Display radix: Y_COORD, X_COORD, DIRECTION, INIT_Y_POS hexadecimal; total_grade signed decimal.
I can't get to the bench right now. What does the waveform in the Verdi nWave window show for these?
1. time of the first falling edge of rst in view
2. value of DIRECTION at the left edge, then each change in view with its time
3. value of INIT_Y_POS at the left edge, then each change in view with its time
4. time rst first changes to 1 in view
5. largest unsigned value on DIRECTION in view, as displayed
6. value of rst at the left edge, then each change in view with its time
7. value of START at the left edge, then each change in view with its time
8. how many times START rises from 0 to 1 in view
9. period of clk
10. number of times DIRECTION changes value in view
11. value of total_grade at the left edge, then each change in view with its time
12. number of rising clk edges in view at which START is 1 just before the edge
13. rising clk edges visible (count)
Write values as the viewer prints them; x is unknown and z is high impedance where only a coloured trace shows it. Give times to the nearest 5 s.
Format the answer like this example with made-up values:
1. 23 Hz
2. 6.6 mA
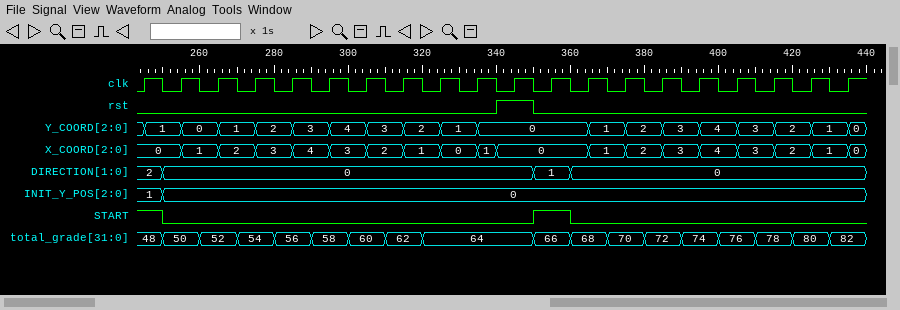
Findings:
1. 350 s
2. 2, 0 at 250 s, 1 at 350 s, 0 at 360 s
3. 1, 0 at 250 s
4. 340 s
5. 2
6. 0, 1 at 340 s, 0 at 350 s
7. 1, 0 at 250 s, 1 at 350 s, 0 at 360 s
8. 1
9. 10 s
10. 3
11. 48, 50 at 250 s, 52 at 260 s, 54 at 270 s, 56 at 280 s, 58 at 290 s, 60 at 300 s, 62 at 310 s, 64 at 320 s, 66 at 350 s, 68 at 360 s, 70 at 370 s, 72 at 380 s, 74 at 390 s, 76 at 400 s, 78 at 410 s, 80 at 420 s, 82 at 430 s
12. 2
13. 20
